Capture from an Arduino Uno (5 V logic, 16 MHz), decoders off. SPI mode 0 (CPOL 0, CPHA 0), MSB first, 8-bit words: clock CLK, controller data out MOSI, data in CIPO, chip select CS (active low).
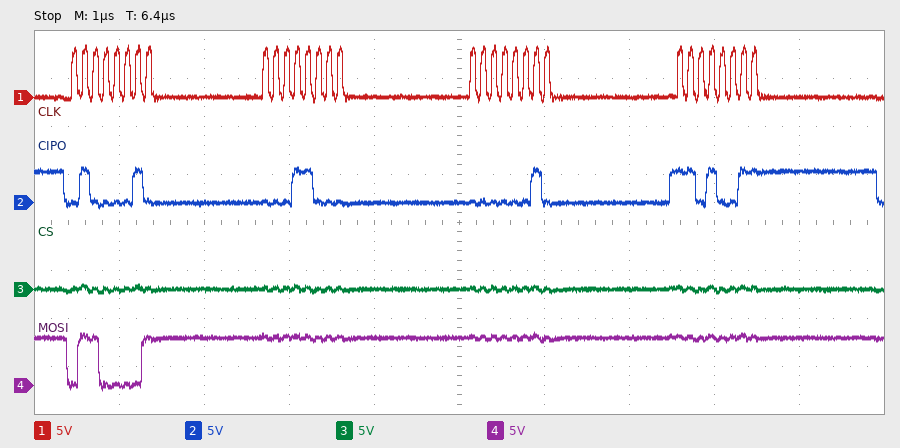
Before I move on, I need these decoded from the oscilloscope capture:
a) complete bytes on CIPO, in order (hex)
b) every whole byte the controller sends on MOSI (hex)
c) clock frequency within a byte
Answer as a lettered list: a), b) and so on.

a) 0x42 0x18 0x02 0xD3
b) 0x61 0xFF 0xFF 0xFF
c) 8 MHz
